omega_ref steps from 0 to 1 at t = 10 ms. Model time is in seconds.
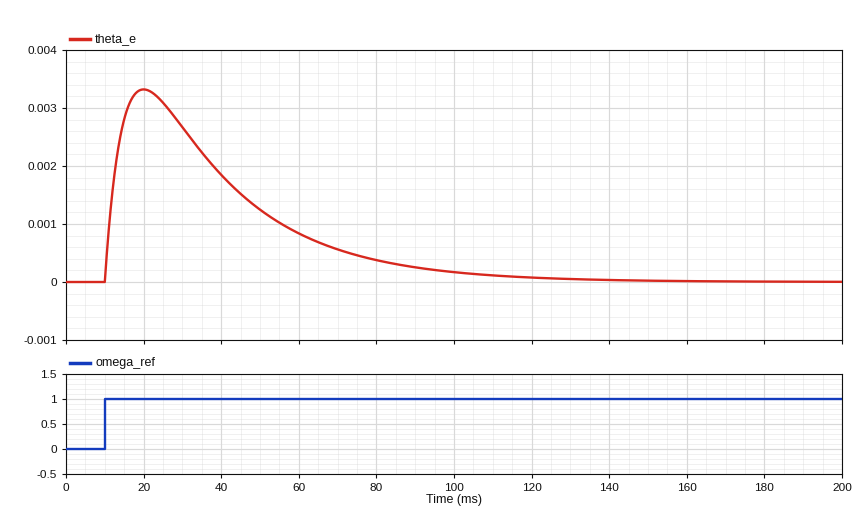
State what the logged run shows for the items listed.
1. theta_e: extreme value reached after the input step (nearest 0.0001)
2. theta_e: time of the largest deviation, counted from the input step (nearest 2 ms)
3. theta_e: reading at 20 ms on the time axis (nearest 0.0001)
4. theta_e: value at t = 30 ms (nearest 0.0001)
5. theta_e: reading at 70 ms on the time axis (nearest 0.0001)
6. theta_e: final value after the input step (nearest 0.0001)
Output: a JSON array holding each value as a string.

["0.0033", "10 ms", "0.0033", "0.0027", "0.0006", "0.0000"]
